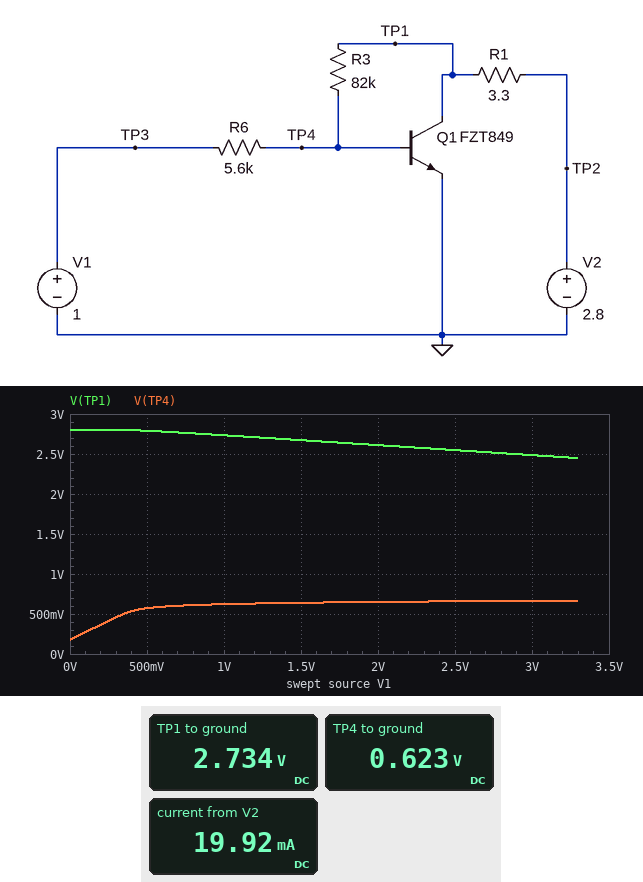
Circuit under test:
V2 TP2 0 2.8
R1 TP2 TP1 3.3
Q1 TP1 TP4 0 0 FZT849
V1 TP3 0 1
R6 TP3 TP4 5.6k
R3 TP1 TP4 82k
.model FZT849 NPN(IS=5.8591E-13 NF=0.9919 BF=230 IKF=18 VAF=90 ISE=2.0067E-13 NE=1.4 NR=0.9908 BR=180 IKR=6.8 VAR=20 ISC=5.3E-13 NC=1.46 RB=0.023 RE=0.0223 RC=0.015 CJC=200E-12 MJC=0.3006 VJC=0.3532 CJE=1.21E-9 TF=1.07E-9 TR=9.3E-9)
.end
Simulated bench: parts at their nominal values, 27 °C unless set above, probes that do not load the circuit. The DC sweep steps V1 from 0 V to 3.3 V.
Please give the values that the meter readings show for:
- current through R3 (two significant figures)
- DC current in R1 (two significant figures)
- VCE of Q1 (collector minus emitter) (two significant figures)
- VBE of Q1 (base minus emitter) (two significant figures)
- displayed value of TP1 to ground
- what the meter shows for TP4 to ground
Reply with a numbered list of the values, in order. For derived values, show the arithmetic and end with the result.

1. (2.734 V - 623 mV) / 82 kΩ = 26 µA
2. (2.8 V - 2.734 V) / 3.3 Ω = 20 mA
3. 2.734 V = 2.7 V
4. 623 mV = 620 mV
5. 2.734 V
6. 0.623 V
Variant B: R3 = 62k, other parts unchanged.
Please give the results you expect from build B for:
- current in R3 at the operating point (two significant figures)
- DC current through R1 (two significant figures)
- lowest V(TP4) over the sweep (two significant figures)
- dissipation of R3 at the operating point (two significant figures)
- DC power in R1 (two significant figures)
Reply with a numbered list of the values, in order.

1. 34 µA
2. 22 mA
3. 230 mV
4. 71 µW
5. 1.5 mW
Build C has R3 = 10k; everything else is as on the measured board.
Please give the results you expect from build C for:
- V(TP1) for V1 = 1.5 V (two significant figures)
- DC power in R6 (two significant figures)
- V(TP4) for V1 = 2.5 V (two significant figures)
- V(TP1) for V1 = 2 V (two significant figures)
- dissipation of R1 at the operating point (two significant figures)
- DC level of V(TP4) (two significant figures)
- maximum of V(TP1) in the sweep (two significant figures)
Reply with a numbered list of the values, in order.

1. 2.6 V
2. 22 µW
3. 670 mV
4. 2.5 V
5. 10 mW
6. 650 mV
7. 2.7 V
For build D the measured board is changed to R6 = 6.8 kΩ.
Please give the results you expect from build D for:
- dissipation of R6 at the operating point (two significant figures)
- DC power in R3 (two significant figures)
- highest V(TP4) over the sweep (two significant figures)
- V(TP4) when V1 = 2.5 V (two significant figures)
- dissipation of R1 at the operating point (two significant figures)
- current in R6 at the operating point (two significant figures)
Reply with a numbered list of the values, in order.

1. 21 µW
2. 55 µW
3. 660 mV
4. 650 mV
5. 1.0 mW
6. 56 µA
